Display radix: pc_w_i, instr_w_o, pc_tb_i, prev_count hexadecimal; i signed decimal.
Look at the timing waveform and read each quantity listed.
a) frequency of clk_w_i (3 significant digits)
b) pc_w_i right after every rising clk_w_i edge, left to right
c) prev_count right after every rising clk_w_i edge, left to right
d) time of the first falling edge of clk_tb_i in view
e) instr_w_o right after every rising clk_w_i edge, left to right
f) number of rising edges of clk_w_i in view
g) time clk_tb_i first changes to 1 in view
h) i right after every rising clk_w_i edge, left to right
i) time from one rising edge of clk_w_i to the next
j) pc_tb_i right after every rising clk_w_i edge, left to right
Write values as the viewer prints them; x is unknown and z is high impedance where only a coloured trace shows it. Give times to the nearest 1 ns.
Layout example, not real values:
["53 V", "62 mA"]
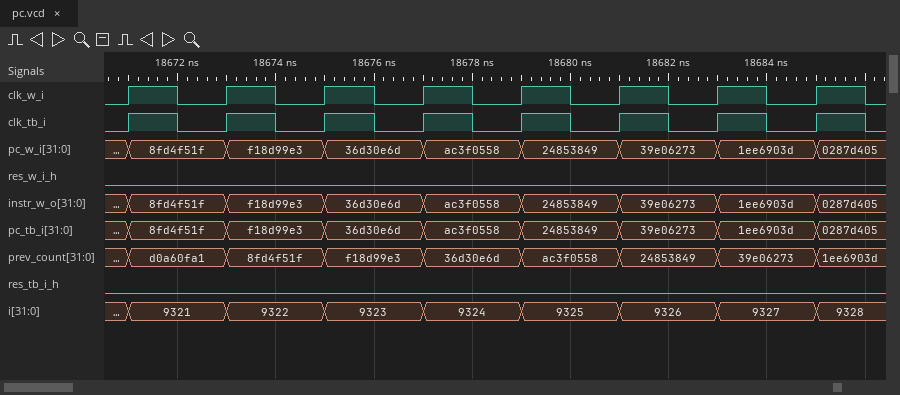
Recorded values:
["500 MHz", "8fd4f51f, f18d99e3, 36d30e6d, ac3f0558, 24853849, 39e06273, 1ee6903d, 0287d405", "d0a60fa1, 8fd4f51f, f18d99e3, 36d30e6d, ac3f0558, 24853849, 39e06273, 1ee6903d", "18672 ns", "8fd4f51f, f18d99e3, 36d30e6d, ac3f0558, 24853849, 39e06273, 1ee6903d, 0287d405", "8", "18671 ns", "9321, 9322, 9323, 9324, 9325, 9326, 9327, 9328", "2 ns", "8fd4f51f, f18d99e3, 36d30e6d, ac3f0558, 24853849, 39e06273, 1ee6903d, 0287d405"]
